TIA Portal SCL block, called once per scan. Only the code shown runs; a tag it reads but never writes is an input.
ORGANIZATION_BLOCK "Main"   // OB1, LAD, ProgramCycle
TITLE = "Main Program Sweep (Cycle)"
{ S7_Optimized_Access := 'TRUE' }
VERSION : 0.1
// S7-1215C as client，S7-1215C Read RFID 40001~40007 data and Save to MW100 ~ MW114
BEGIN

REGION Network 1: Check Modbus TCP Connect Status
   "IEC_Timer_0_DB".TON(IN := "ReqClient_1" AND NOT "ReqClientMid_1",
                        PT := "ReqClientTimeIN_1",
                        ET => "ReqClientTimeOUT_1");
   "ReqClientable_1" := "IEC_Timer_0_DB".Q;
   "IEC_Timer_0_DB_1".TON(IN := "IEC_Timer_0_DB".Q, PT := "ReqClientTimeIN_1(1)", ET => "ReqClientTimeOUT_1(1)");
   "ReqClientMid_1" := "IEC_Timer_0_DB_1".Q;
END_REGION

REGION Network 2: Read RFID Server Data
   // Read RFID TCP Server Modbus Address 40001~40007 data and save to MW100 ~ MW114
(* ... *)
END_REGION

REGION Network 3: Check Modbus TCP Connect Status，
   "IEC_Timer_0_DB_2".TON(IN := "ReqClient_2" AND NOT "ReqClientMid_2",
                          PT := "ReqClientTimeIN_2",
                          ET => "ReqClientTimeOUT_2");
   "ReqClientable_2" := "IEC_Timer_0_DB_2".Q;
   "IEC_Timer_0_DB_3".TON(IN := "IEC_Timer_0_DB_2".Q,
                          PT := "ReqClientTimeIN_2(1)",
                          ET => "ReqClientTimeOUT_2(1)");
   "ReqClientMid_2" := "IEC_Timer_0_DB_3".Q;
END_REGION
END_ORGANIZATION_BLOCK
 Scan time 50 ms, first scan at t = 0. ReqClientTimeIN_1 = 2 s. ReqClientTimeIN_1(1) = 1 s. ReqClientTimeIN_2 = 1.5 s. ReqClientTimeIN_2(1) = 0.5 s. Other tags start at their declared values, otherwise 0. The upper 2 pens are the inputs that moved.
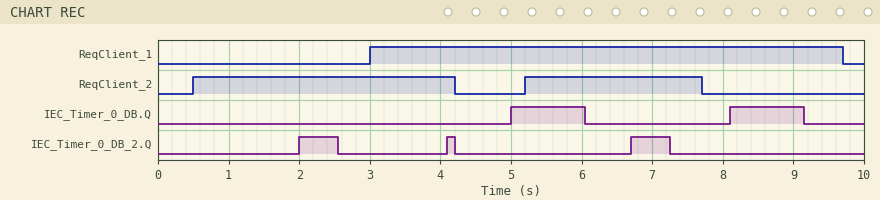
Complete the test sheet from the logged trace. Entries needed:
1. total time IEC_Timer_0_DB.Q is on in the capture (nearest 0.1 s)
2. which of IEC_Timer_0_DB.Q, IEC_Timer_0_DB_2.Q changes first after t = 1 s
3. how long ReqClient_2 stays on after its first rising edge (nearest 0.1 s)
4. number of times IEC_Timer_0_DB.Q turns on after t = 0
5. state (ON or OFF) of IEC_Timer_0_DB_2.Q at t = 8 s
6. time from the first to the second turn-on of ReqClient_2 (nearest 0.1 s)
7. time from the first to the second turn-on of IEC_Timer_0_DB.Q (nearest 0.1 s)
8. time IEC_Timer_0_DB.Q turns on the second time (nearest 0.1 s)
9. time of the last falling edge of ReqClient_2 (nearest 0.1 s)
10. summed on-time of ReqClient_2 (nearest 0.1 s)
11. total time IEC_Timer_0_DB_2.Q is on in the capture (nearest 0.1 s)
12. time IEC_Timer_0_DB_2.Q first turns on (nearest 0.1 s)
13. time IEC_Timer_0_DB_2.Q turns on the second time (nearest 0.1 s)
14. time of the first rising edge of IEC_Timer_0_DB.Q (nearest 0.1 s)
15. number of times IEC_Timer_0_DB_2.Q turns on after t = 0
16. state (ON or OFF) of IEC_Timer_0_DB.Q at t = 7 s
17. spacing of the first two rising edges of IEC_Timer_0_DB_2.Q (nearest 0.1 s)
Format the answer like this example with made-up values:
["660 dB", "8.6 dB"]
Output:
["2.1 s", "IEC_Timer_0_DB_2.Q", "3.7 s", "2", "OFF", "4.7 s", "3.1 s", "8.1 s", "7.7 s", "6.2 s", "1.2 s", "2.0 s", "4.1 s", "5.0 s", "3", "OFF", "2.1 s"]
